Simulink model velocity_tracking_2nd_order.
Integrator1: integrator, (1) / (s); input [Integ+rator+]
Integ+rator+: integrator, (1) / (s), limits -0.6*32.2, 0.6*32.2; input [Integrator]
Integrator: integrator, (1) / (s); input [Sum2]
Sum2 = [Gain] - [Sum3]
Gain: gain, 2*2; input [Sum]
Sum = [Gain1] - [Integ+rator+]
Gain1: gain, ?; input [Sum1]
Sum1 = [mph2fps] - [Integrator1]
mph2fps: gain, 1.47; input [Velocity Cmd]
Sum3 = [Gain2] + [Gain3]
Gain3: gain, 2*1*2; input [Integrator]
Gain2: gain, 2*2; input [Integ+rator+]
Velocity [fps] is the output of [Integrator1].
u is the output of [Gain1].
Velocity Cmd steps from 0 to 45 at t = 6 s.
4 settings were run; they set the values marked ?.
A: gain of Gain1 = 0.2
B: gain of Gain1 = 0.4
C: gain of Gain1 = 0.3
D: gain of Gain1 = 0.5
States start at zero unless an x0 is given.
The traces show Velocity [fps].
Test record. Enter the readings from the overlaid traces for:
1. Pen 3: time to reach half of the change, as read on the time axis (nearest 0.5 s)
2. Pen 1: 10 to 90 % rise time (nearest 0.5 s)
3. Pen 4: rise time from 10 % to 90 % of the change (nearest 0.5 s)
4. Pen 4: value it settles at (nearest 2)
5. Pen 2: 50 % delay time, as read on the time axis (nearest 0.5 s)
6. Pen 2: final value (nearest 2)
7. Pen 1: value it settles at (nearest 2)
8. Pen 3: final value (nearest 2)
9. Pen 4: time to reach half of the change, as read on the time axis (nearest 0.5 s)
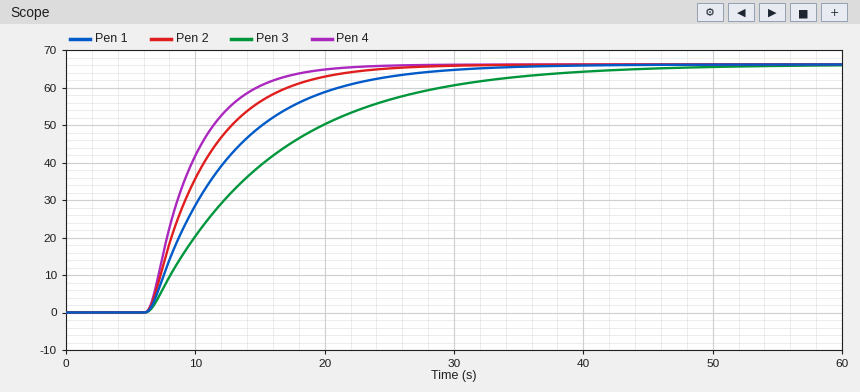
13.0 s
13.5 s
7.5 s
66
9.5 s
66
66
66
9.0 s
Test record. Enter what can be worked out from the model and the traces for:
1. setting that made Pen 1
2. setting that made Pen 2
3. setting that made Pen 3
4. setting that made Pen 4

C
B
A
D
